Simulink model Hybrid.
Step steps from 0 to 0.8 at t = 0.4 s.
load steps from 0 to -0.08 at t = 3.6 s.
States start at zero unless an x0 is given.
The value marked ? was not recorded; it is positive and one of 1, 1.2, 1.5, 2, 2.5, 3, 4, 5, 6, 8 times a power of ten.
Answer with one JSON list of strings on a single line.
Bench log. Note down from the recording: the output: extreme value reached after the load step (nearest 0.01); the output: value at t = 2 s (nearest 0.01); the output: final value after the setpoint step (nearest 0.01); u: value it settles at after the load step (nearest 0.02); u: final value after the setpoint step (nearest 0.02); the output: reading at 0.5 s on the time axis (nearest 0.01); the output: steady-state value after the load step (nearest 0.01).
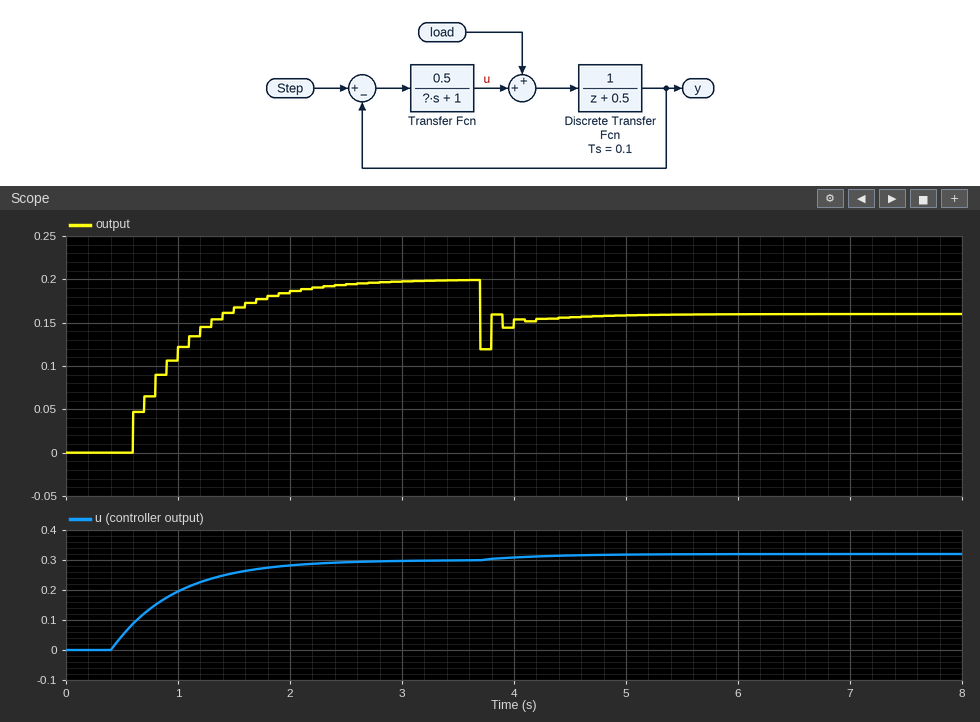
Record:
["0.12", "0.19", "0.20", "0.32", "0.30", "0.00", "0.16"]
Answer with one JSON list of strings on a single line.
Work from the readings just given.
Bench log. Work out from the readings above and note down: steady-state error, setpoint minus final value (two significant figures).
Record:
["0.60"]
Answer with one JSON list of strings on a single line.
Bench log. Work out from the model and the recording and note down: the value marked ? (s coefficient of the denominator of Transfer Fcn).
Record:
["0.8"]
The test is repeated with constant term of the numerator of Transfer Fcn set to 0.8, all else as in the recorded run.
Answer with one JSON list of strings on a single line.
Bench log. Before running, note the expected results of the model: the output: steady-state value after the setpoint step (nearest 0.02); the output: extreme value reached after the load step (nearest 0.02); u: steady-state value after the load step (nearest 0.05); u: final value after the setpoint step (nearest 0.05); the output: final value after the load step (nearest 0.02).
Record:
["0.28", "0.20", "0.45", "0.40", "0.24"]
